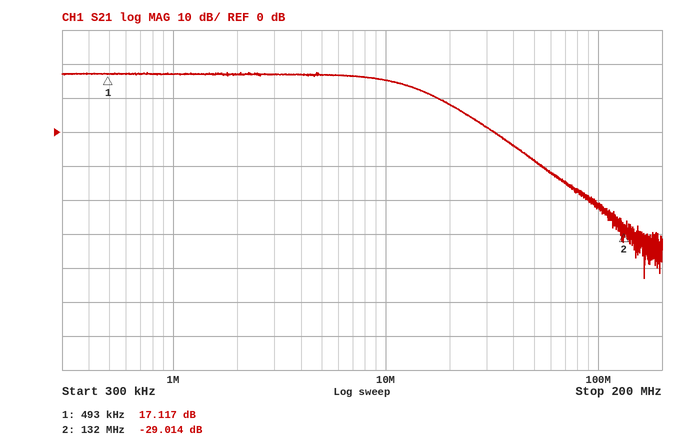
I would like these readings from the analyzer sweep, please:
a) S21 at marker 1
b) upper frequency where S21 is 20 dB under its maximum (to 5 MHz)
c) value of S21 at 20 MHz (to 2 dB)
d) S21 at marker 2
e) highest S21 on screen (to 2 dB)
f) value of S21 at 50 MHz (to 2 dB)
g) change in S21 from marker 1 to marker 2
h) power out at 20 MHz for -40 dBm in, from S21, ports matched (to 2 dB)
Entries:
17.117 dB
35 MHz
8 dB
-29.014 dB
18 dB
-8 dB
-46.131 dB
-32 dBm
